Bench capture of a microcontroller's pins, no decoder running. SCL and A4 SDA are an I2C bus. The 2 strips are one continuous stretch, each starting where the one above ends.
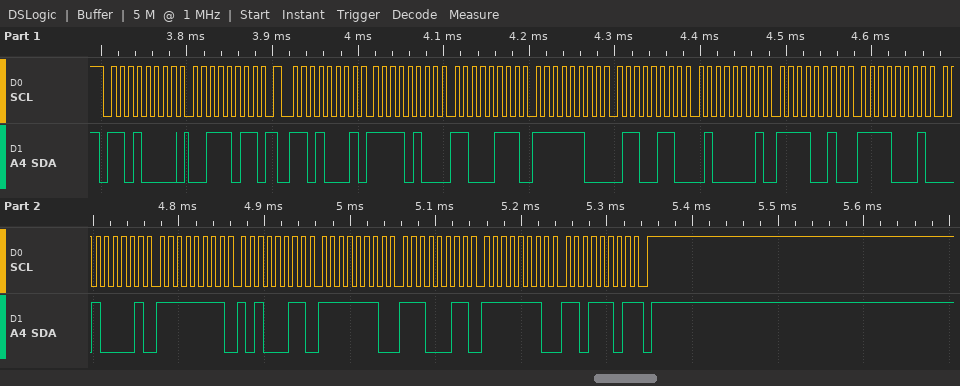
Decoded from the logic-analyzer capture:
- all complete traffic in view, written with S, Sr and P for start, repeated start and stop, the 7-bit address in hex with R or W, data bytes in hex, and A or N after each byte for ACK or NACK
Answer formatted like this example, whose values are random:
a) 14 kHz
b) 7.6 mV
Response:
a) S 68W A 3B A Sr 68R A F4 A C7 A FC A 66 A 41 A F2 A F1 A 21 A FF A A3 A FE A E3 A FE A DD N P
